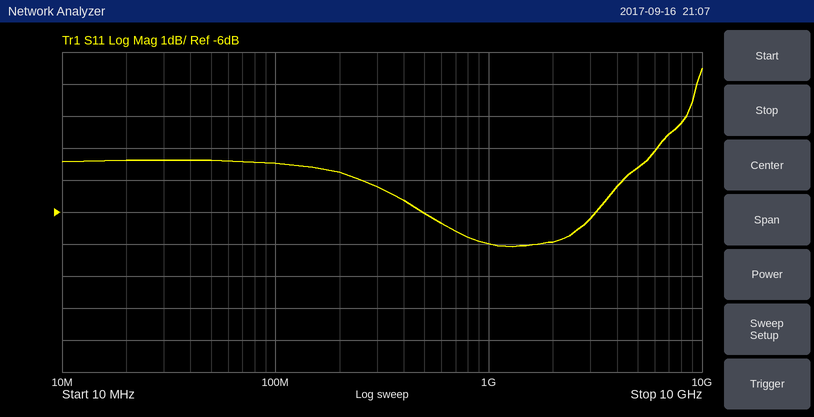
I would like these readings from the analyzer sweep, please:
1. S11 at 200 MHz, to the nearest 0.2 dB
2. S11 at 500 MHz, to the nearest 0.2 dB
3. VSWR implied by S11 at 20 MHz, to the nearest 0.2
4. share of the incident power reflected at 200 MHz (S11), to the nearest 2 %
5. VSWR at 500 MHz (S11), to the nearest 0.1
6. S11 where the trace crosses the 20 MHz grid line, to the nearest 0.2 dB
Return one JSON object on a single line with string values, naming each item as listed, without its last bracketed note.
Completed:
{"S11 at 200 MHz, to the nearest 0.2 dB": "-4.8 dB", "S11 at 500 MHz, to the nearest 0.2 dB": "-6.0 dB", "VSWR implied by S11 at 20 MHz, to the nearest 0.2": "4.0", "share of the incident power reflected at 200 MHz (S11), to the nearest 2 %": "34 %", "VSWR at 500 MHz (S11), to the nearest 0.1": "3.0", "S11 where the trace crosses the 20 MHz grid line, to the nearest 0.2 dB": "-4.4 dB"}
